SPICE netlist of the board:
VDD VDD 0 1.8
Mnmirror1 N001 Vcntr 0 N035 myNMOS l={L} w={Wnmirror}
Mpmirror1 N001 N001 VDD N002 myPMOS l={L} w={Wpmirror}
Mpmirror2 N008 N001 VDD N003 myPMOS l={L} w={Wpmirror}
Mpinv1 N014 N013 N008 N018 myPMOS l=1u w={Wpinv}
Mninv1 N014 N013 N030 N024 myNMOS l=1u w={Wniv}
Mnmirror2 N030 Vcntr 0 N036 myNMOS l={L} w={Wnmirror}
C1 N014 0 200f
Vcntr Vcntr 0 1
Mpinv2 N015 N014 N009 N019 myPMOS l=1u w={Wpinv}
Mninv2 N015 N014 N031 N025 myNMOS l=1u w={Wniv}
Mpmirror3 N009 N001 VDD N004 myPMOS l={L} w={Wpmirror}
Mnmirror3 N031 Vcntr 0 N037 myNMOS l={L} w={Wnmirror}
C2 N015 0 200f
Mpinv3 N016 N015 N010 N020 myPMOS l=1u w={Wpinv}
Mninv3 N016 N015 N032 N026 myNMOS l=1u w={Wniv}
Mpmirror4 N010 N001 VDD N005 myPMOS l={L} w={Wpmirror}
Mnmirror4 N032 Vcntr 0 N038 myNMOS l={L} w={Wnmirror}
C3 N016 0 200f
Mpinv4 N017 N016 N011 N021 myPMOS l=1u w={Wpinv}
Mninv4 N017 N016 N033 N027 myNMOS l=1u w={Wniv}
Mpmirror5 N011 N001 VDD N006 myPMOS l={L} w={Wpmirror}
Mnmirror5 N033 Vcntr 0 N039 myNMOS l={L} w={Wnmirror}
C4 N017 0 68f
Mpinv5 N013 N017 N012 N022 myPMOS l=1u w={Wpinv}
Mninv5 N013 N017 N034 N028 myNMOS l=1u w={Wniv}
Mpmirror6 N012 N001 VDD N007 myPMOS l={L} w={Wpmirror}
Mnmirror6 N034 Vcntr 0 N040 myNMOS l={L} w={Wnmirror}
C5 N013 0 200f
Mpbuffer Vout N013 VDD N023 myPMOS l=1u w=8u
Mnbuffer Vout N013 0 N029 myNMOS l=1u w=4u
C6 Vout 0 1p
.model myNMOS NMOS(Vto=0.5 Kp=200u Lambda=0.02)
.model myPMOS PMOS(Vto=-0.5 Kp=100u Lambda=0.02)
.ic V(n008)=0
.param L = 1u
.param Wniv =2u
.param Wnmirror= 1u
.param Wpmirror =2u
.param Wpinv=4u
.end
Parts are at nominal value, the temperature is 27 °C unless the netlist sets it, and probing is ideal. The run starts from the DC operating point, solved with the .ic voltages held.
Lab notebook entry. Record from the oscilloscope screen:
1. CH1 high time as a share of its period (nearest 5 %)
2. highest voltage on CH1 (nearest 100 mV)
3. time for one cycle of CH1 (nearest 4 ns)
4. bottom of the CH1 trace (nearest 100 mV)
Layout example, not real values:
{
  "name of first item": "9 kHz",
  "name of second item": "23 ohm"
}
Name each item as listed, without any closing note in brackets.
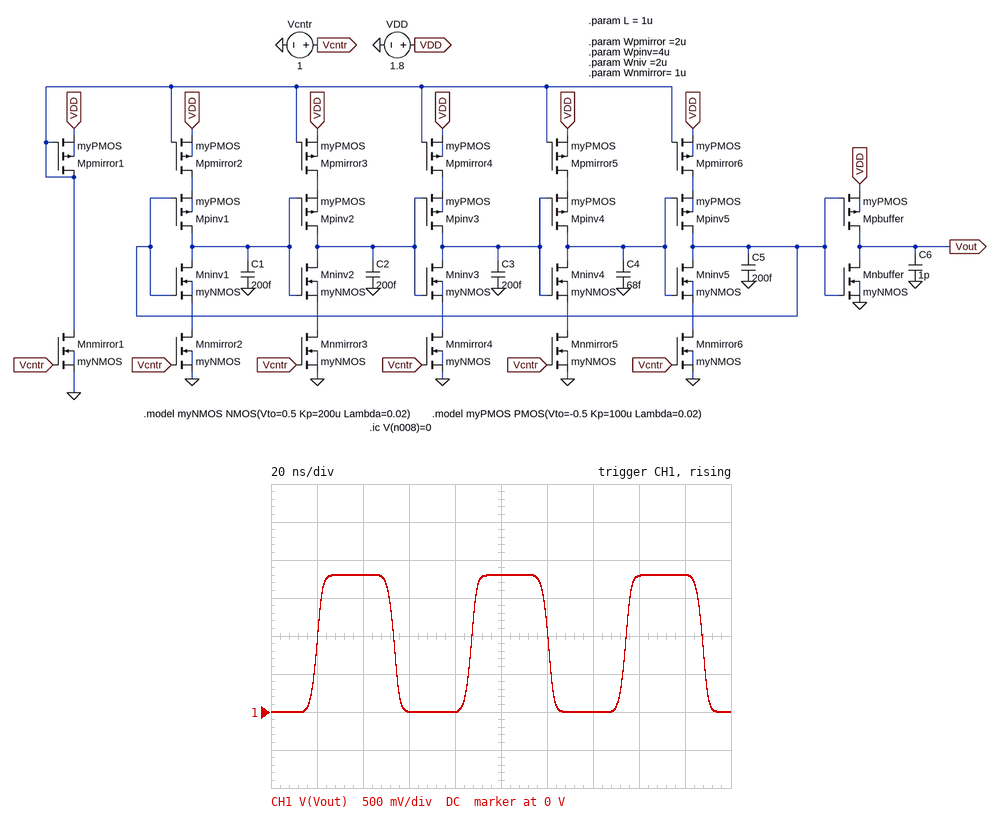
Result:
{
  "CH1 high time as a share of its period": "50 %",
  "highest voltage on CH1": "1.8 V",
  "time for one cycle of CH1": "68 ns",
  "bottom of the CH1 trace": "0 V"
}
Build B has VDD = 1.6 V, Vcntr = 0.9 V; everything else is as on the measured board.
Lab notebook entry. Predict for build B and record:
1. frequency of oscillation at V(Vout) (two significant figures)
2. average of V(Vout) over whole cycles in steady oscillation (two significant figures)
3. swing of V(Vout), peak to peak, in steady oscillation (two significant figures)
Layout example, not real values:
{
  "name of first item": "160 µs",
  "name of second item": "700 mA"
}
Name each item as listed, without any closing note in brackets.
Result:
{
  "frequency of oscillation at V(Vout)": "11 MHz",
  "average of V(Vout) over whole cycles in steady oscillation": "800 mV",
  "swing of V(Vout), peak to peak, in steady oscillation": "1.6 V"
}
